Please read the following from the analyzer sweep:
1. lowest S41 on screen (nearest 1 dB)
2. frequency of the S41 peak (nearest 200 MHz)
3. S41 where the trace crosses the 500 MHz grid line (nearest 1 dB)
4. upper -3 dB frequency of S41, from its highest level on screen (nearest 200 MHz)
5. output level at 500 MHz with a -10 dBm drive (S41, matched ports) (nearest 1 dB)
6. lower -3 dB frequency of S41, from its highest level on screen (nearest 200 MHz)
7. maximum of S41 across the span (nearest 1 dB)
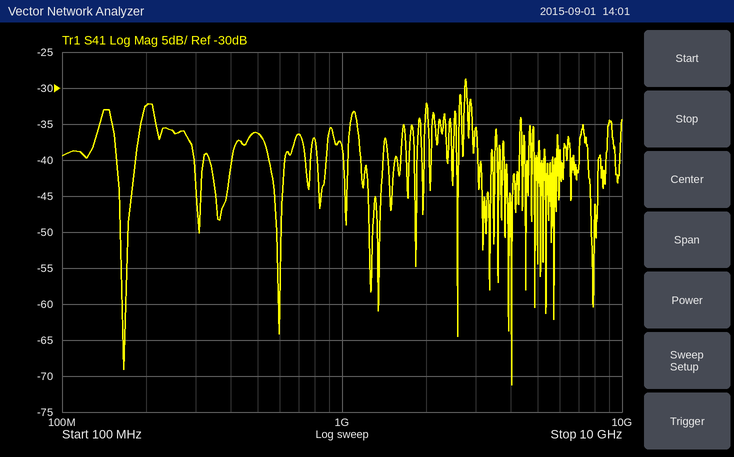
-71 dB
2.8 GHz
-36 dB
2.8 GHz
-46 dBm
2.8 GHz
-29 dB
